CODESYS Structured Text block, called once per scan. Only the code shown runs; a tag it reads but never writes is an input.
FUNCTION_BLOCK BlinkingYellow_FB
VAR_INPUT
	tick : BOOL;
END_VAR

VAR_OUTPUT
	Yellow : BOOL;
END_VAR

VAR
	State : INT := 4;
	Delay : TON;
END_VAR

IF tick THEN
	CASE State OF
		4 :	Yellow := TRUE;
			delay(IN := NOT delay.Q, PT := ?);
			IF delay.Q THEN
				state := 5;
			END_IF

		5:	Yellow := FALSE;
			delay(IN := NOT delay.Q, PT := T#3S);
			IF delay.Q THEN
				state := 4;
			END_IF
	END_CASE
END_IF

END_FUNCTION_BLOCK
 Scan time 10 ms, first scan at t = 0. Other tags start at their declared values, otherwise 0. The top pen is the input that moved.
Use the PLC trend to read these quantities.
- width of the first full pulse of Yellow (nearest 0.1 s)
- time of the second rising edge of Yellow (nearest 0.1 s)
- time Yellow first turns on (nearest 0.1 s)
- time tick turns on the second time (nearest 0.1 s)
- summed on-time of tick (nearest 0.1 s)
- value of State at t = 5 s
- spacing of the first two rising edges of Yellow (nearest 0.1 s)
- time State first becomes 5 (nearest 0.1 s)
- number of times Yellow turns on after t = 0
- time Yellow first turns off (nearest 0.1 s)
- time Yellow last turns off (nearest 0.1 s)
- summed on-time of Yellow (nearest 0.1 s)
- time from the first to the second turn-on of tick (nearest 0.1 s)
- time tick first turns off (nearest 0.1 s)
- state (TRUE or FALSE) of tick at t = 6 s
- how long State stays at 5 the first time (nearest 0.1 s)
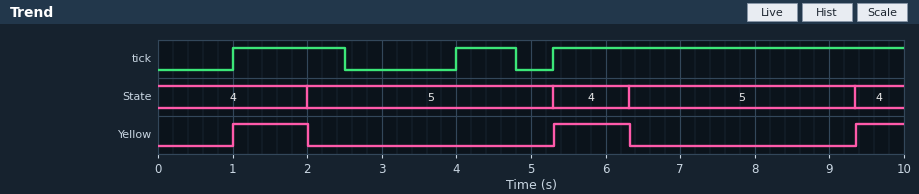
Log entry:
1.0 s
5.3 s
1.0 s
4.0 s
7.0 s
5
4.3 s
2.0 s
3
2.0 s
6.3 s
2.7 s
3.0 s
2.5 s
TRUE
3.3 s
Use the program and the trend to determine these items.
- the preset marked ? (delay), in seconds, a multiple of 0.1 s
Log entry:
1.0 s
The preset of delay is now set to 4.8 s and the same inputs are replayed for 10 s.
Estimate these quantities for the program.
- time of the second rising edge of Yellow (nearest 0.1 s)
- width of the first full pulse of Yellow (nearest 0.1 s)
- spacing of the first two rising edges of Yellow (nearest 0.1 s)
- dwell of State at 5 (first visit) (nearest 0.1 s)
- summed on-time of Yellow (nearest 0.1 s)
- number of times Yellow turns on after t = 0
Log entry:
8.8 s
4.8 s
7.8 s
3.0 s
6.0 s
2
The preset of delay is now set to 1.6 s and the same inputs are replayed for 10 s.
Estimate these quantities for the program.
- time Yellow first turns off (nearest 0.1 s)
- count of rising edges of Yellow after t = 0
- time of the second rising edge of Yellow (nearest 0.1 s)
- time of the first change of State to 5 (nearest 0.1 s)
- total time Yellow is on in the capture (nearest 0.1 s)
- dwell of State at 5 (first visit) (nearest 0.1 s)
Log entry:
4.0 s
2
7.0 s
4.0 s
4.6 s
3.0 s
